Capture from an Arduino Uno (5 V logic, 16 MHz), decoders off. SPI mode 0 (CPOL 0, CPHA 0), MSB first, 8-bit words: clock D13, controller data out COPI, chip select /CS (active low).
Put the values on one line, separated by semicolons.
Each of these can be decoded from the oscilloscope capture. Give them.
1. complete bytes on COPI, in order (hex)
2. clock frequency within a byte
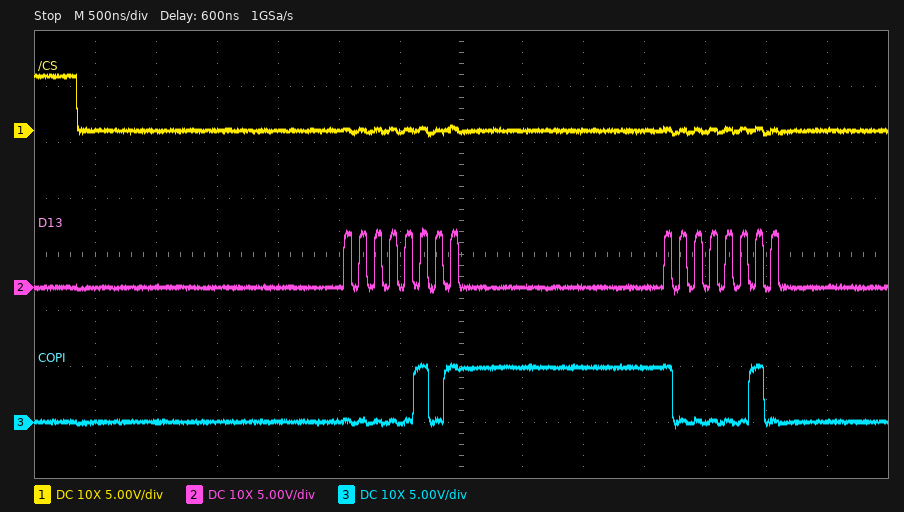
05 82; 8 MHz
